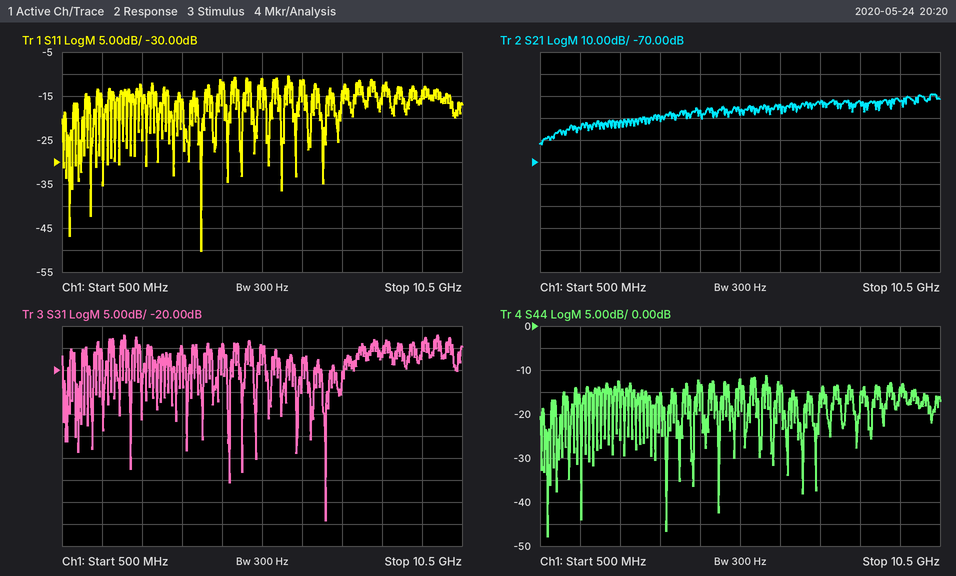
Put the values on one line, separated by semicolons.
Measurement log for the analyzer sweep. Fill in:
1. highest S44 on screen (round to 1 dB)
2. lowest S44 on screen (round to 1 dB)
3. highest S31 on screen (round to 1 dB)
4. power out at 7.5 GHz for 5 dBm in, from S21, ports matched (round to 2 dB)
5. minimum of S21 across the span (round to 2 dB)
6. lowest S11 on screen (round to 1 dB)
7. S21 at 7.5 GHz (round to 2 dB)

-11 dB; -48 dB; -12 dB; -38 dBm; -62 dB; -50 dB; -44 dB
